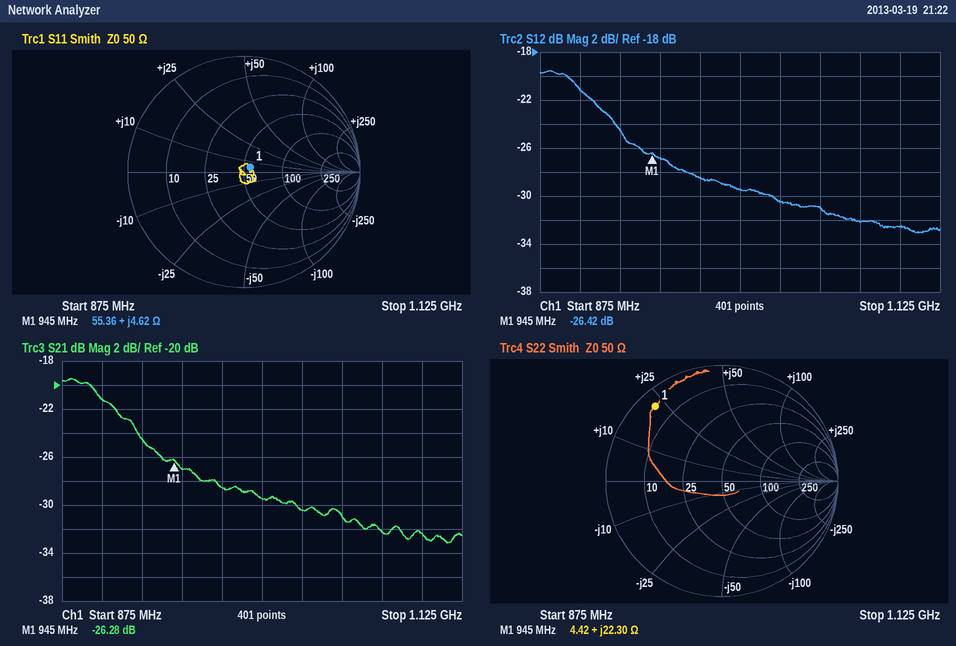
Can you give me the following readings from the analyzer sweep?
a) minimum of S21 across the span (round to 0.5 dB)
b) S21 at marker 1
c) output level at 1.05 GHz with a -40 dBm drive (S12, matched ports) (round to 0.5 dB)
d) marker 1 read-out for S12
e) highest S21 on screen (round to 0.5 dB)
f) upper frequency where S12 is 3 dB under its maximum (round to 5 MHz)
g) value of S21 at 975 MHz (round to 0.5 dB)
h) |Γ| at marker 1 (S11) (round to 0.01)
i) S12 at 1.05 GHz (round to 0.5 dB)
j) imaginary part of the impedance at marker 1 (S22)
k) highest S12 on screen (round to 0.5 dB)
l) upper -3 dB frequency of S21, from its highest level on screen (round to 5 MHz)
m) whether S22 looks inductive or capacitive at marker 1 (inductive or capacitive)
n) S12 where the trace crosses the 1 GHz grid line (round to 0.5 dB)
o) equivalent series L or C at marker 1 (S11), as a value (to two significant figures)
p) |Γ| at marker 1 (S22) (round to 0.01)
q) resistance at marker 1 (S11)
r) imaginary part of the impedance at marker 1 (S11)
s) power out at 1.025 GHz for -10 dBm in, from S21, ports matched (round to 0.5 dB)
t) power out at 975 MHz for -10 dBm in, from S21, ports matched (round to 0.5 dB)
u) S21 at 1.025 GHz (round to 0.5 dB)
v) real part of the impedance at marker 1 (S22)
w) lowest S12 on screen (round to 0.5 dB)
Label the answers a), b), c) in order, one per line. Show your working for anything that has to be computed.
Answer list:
a) -33.0 dB
b) -26.28 dB
c) -40 dBm + (-31.0 dB) = -71.0 dBm
d) -26.42 dB
e) -19.5 dB
f) 910 MHz
g) -28.5 dB
h) 0.07
i) -31.0 dB
j) +22.30 Ω
k) -19.5 dB
l) 910 MHz
m) inductive
n) -29.5 dB
o) L = 4.62 Ω/(2π × 945 MHz) ≈ 778 pH, so 780 pH to two significant figures
p) 0.86
q) 55.36 Ω
r) +4.62 Ω
s) -10 dBm + (-30.5 dB) = -40.5 dBm
t) -10 dBm + (-28.5 dB) = -38.5 dBm
u) -30.5 dB
v) 4.42 Ω
w) -33.0 dB
